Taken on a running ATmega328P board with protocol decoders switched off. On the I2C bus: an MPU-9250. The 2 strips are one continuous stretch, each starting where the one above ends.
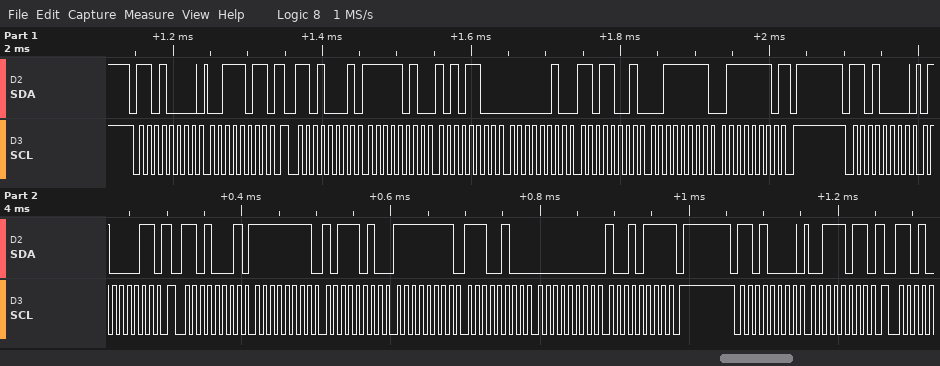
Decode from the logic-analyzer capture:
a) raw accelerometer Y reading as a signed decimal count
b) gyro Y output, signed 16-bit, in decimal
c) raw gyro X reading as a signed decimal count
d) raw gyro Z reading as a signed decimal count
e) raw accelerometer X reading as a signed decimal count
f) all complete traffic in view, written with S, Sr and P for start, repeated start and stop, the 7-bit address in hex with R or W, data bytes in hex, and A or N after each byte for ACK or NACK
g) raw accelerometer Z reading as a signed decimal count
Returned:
729
-28
-70
151
-1364
S 68W A 3B A Sr 68R A FA A AC A 02 A D9 A 3F A 7E N P S 68W A 43 A Sr 68R A FF A BA A FF A E4 A 00 A 97 N P S 68W A 3B A
16254
